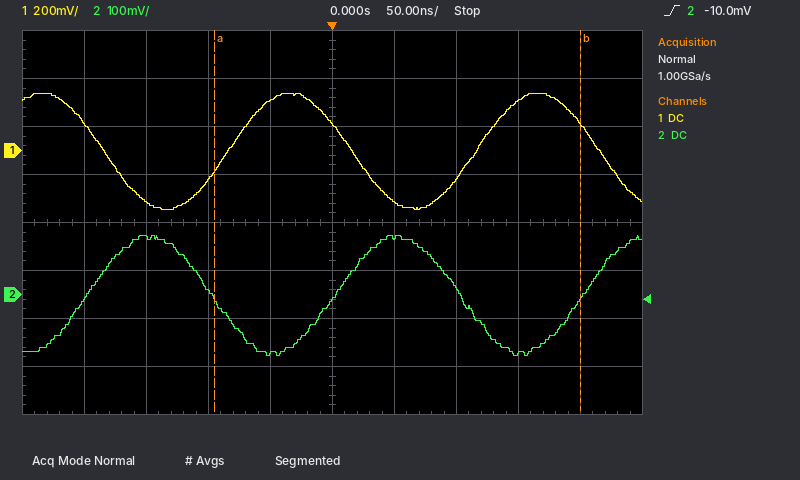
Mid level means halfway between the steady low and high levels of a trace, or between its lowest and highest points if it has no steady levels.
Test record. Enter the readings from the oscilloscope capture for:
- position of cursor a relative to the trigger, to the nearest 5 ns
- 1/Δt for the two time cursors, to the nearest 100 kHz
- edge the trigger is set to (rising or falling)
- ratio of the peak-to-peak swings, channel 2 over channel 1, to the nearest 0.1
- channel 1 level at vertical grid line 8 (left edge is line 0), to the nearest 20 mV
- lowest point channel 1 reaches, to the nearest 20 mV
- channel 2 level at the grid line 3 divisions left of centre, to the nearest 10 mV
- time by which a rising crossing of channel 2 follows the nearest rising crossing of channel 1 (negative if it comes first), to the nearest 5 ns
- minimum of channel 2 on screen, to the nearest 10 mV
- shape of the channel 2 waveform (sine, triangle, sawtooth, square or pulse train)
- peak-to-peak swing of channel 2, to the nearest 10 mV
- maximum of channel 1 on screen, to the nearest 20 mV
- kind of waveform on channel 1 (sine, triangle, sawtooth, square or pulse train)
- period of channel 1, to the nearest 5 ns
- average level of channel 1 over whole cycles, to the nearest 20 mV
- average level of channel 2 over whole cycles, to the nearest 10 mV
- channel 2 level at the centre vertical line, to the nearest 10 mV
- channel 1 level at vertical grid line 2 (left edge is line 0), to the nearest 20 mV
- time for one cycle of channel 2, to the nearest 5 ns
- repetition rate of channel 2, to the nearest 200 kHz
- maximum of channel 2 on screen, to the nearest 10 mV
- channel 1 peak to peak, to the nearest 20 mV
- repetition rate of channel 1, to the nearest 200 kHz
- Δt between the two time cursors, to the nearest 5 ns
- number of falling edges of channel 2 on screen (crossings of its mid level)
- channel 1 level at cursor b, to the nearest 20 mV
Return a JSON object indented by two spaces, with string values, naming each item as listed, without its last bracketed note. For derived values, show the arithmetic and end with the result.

{
  "position of cursor a relative to the trigger, to the nearest 5 ns": "-95 ns",
  "1/Δt for the two time cursors, to the nearest 100 kHz": "1 / 295 ns ≈ 3.4 MHz",
  "edge the trigger is set to": "rising",
  "ratio of the peak-to-peak swings, channel 2 over channel 1, to the nearest 0.1": "250 mV / 480 mV ≈ 0.5",
  "channel 1 level at vertical grid line 8 (left edge is line 0), to the nearest 20 mV": "200 mV",
  "lowest point channel 1 reaches, to the nearest 20 mV": "-240 mV",
  "channel 2 level at the grid line 3 divisions left of centre, to the nearest 10 mV": "120 mV",
  "time by which a rising crossing of channel 2 follows the nearest rising crossing of channel 1 (negative if it comes first), to the nearest 5 ns": "+85 ns",
  "minimum of channel 2 on screen, to the nearest 10 mV": "-130 mV",
  "shape of the channel 2 waveform": "sine",
  "peak-to-peak swing of channel 2, to the nearest 10 mV": "120 mV − (-130 mV) = 250 mV",
  "maximum of channel 1 on screen, to the nearest 20 mV": "240 mV",
  "kind of waveform on channel 1": "sine",
  "period of channel 1, to the nearest 5 ns": "200 ns",
  "average level of channel 1 over whole cycles, to the nearest 20 mV": "(240 mV + (-240 mV)) / 2 ≈ 0 mV",
  "average level of channel 2 over whole cycles, to the nearest 10 mV": "(120 mV + (-130 mV)) / 2 ≈ 0 mV",
  "channel 2 level at the centre vertical line, to the nearest 10 mV": "-10 mV",
  "channel 1 level at vertical grid line 2 (left edge is line 0), to the nearest 20 mV": "-220 mV",
  "time for one cycle of channel 2, to the nearest 5 ns": "200 ns",
  "repetition rate of channel 2, to the nearest 200 kHz": "1 / 200 ns ≈ 5.0 MHz",
  "maximum of channel 2 on screen, to the nearest 10 mV": "120 mV",
  "channel 1 peak to peak, to the nearest 20 mV": "240 mV − (-240 mV) = 480 mV",
  "repetition rate of channel 1, to the nearest 200 kHz": "1 / 200 ns ≈ 5.0 MHz",
  "Δt between the two time cursors, to the nearest 5 ns": "295 ns",
  "number of falling edges of channel 2 on screen": "2",
  "channel 1 level at cursor b, to the nearest 20 mV": "120 mV"
}
